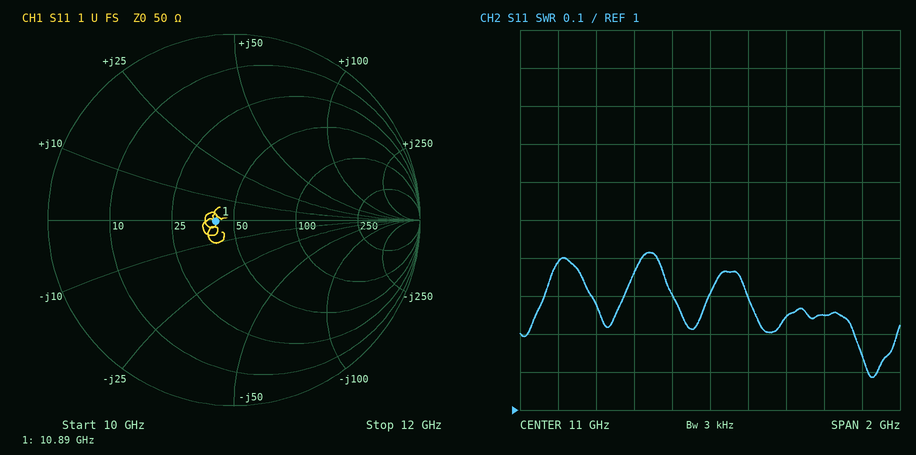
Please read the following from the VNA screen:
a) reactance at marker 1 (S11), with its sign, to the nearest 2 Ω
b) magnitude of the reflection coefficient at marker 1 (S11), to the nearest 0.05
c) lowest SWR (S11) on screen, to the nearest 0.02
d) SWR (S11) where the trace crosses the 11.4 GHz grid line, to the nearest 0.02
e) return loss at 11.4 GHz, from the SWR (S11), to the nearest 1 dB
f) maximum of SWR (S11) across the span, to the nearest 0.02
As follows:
0 Ω
0.10
1.08
1.24
19 dB
1.42
